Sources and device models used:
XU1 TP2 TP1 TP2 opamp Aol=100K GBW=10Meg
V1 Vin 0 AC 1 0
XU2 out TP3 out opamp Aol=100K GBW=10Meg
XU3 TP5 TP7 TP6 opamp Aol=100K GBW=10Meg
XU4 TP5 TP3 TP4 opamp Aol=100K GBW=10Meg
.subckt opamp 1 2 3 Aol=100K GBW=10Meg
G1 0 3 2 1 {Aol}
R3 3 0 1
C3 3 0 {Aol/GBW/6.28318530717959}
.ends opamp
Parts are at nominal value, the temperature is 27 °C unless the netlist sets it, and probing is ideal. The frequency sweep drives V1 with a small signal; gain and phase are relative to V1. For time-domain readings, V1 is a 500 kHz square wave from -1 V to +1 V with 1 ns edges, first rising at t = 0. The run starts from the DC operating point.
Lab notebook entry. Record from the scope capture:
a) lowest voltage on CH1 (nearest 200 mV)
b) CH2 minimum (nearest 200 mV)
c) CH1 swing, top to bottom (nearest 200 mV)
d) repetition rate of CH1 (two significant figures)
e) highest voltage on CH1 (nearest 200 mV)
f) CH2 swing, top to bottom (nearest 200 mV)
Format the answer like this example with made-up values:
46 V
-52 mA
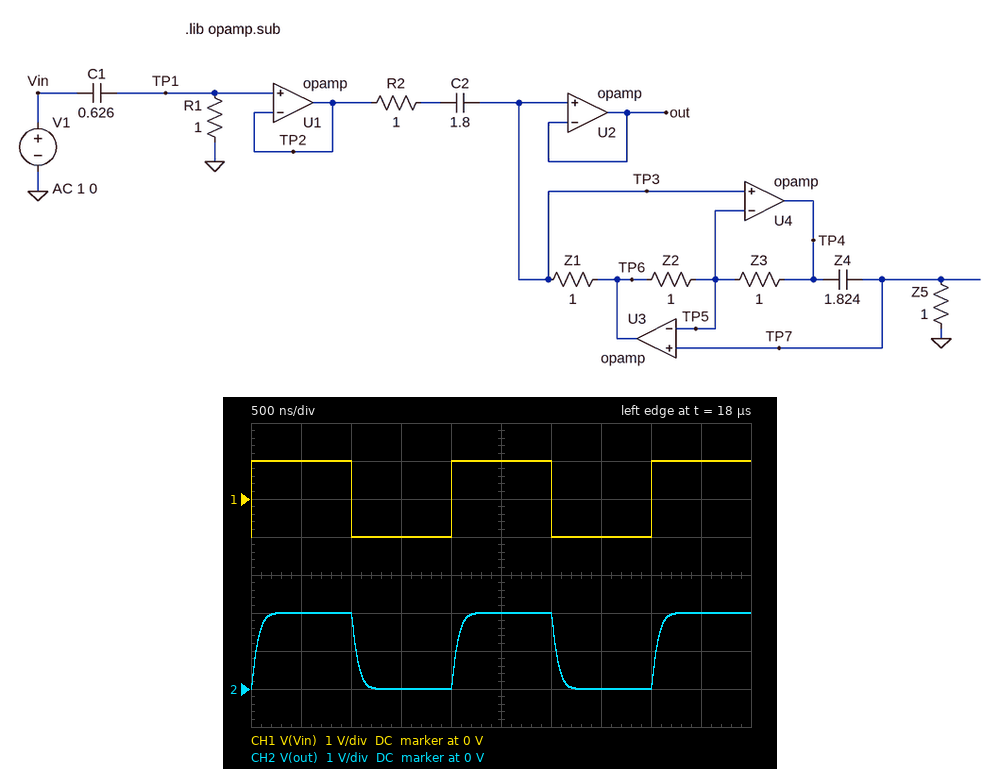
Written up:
-1.0 V
0 V
2.0 V
500 kHz
1.0 V
2.0 V
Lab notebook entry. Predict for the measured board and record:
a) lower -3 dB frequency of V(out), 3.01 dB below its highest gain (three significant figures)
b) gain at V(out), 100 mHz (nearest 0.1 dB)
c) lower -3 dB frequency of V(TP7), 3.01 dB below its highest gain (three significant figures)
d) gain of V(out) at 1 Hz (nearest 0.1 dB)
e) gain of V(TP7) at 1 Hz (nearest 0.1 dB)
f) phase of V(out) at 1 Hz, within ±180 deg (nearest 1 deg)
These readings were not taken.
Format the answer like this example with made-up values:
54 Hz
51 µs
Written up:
222 mHz
-7.8 dB
222 mHz
-0.2 dB
-0.2 dB
19 deg
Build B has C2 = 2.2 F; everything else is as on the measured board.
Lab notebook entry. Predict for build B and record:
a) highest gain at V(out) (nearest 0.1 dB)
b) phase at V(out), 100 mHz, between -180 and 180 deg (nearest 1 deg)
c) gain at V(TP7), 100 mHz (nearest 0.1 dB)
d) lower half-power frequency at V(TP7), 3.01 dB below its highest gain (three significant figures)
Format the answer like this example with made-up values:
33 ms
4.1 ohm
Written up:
0 dB
136 deg
-8.3 dB
235 mHz
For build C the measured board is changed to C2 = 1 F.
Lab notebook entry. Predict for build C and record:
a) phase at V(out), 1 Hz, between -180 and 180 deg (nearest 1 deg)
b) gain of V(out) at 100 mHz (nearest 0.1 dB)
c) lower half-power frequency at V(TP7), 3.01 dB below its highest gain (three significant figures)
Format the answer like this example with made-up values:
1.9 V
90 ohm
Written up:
19 deg
-8.3 dB
142 mHz
